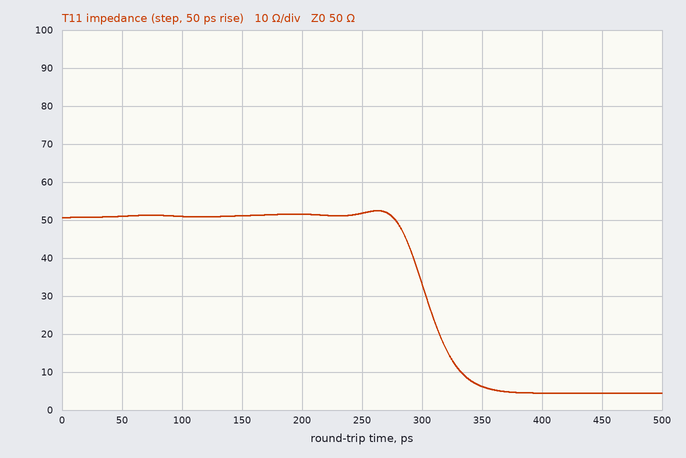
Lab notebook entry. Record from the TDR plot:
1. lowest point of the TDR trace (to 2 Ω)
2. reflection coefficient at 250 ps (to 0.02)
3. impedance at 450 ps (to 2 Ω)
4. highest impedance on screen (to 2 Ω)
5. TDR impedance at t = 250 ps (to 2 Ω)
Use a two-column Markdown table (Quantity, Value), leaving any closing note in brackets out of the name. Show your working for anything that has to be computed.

| Quantity | Value |
|---|---|
| lowest point of the TDR trace | 4 Ω |
| reflection coefficient at 250 ps | (52 − 50)/(52 + 50) ≈ +0.02 |
| impedance at 450 ps | 4 Ω |
| highest impedance on screen | 52 Ω |
| TDR impedance at t = 250 ps | 52 Ω |
